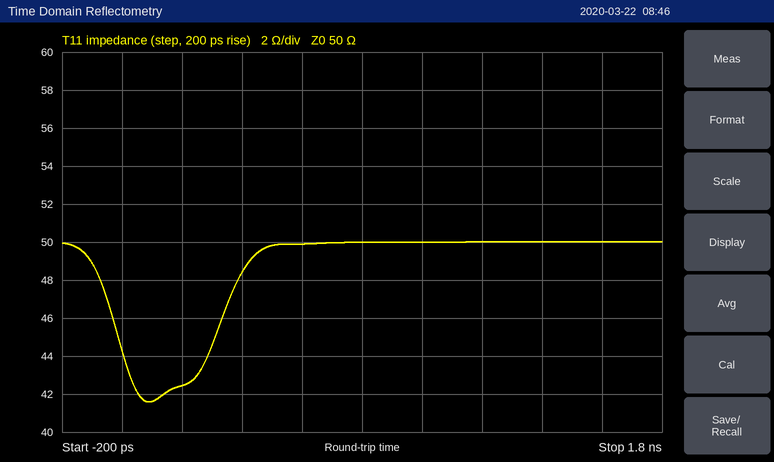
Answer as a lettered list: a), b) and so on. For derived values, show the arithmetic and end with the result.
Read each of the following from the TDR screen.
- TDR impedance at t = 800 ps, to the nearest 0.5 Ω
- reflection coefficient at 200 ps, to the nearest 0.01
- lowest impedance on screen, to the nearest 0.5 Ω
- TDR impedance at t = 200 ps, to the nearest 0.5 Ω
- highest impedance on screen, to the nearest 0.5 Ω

a) 50.0 Ω
b) (42.5 − 50)/(42.5 + 50) ≈ -0.08
c) 41.5 Ω
d) 42.5 Ω
e) 50.0 Ω
